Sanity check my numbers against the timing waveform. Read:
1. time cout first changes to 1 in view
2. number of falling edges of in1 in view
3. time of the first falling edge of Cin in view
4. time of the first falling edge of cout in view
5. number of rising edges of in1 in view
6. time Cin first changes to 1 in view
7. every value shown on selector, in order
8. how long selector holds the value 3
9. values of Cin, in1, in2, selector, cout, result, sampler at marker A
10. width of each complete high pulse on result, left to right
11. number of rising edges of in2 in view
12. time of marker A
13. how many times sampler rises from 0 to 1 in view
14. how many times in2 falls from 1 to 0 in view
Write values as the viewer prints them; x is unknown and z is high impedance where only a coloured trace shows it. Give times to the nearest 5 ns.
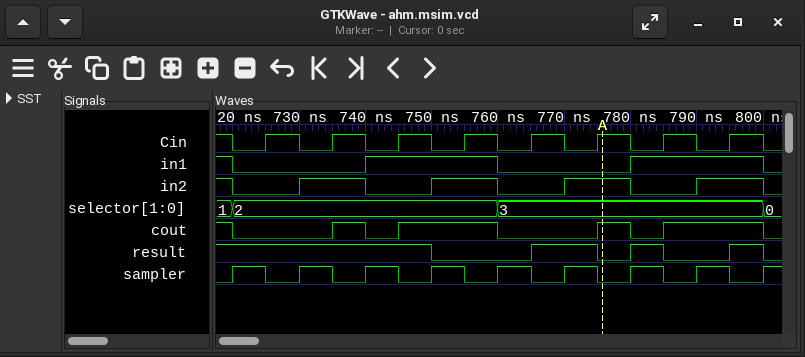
735 ns
3
720 ns
720 ns
2
725 ns
1, 2, 3, 0
40 ns
Cin=1, in1=0, in2=1, selector=3, cout=1, result=0, sampler=0
10 ns, 5 ns, 5 ns
4
775 ns
9
5
